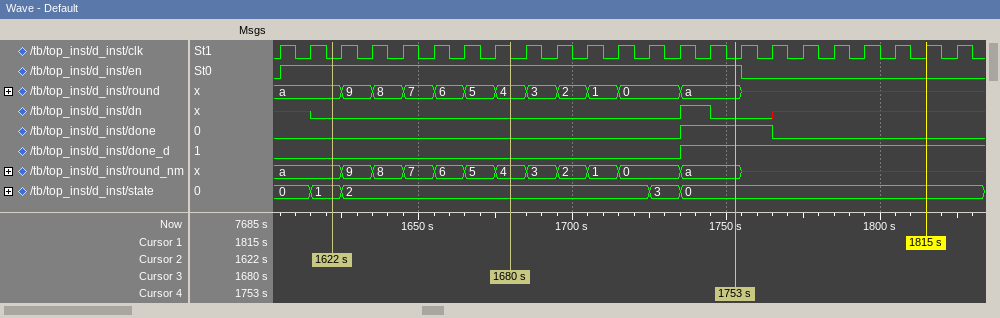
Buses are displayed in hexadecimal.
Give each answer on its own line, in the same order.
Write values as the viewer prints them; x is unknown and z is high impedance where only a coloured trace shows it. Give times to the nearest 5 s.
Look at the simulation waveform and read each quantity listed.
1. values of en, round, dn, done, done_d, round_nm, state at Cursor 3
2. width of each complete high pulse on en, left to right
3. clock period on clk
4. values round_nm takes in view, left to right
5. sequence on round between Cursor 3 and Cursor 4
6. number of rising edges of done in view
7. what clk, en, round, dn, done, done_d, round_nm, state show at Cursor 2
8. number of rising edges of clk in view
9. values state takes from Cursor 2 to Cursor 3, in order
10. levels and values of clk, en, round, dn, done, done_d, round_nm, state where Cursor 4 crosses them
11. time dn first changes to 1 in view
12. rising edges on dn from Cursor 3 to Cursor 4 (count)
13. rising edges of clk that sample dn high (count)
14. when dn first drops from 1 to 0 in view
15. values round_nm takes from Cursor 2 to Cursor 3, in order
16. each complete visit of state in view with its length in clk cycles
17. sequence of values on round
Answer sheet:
en=1, round=4, dn=0, done=0, done_d=0, round_nm=4, state=2
150 s
10 s
a, 9, 8, 7, 6, 5, 4, 3, 2, 1, 0, a, x
4, 3, 2, 1, 0, a
1
clk=0, en=1, round=a, dn=0, done=0, done_d=0, round_nm=a, state=1
23
1, 2
clk=0, en=1, round=a, dn=0, done=1, done_d=1, round_nm=a, state=0
1735 s
1
1
1745 s
a, 9, 8, 7, 6, 5, 4
1: 1, 2: 10, 3: 1
a, 9, 8, 7, 6, 5, 4, 3, 2, 1, 0, a, x
